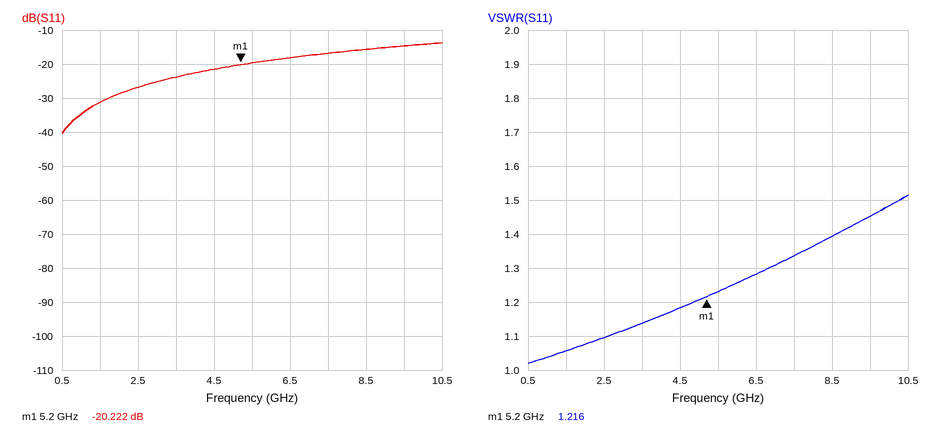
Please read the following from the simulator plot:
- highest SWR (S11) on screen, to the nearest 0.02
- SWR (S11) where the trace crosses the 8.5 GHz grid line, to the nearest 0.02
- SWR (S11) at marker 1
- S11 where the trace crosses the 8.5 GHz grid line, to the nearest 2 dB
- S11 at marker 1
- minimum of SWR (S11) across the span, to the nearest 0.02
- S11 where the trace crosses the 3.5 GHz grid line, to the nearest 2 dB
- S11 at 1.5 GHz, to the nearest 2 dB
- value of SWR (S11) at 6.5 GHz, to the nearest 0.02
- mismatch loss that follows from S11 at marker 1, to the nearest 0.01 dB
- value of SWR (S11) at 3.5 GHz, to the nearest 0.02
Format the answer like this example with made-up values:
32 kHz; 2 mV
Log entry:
1.52; 1.40; 1.216; -16 dB; -20.222 dB; 1.02; -24 dB; -32 dB; 1.28; 0.04 dB; 1.14
